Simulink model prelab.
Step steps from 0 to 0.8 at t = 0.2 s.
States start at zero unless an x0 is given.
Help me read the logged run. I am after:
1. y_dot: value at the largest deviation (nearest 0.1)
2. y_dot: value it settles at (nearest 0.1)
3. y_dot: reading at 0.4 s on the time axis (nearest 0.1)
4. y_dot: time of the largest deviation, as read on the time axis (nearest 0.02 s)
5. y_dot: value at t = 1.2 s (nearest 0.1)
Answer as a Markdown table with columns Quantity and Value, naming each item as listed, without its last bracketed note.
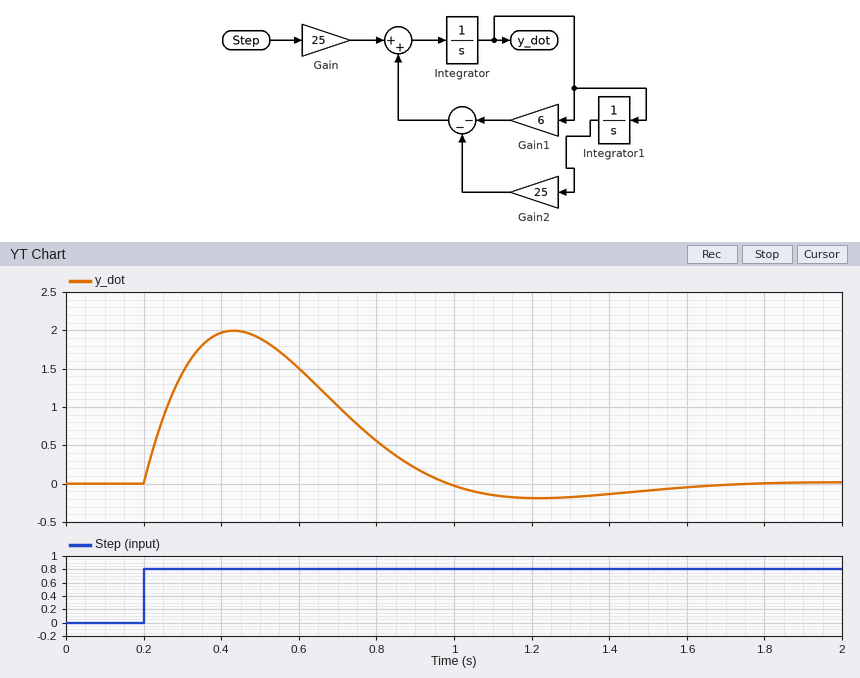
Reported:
| Quantity | Value |
|---|---|
| y_dot: value at the largest deviation | 2.0 |
| y_dot: value it settles at | 0.0 |
| y_dot: reading at 0.4 s on the time axis | 2.0 |
| y_dot: time of the largest deviation, as read on the time axis | 0.44 s |
| y_dot: value at t = 1.2 s | -0.2 |
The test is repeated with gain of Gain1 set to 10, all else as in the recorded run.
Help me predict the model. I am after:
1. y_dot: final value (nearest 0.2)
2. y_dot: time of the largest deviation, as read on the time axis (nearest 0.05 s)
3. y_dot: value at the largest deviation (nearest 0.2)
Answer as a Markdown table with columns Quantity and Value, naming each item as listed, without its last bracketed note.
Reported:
| Quantity | Value |
|---|---|
| y_dot: final value | 0.0 |
| y_dot: time of the largest deviation, as read on the time axis | 0.40 s |
| y_dot: value at the largest deviation | 1.4 |
